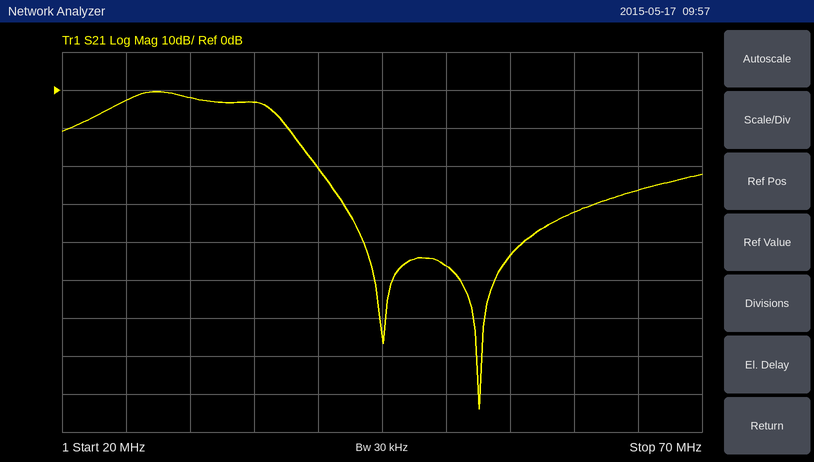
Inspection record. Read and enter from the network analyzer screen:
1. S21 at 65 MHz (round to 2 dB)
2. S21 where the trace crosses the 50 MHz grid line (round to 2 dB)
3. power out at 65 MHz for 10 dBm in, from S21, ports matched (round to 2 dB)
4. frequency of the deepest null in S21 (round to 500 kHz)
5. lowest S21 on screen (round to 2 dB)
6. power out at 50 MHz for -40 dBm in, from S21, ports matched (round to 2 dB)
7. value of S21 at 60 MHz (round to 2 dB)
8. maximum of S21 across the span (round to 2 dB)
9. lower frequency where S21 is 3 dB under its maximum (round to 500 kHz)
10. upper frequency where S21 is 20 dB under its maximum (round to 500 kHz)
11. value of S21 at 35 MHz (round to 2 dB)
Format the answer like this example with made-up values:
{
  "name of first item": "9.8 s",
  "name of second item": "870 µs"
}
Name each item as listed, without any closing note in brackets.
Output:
{
  "S21 at 65 MHz": "-26 dB",
  "S21 where the trace crosses the 50 MHz grid line": "-46 dB",
  "power out at 65 MHz for 10 dBm in, from S21, ports matched": "-16 dBm",
  "frequency of the deepest null in S21": "52.5 MHz",
  "lowest S21 on screen": "-84 dB",
  "power out at 50 MHz for -40 dBm in, from S21, ports matched": "-86 dBm",
  "value of S21 at 60 MHz": "-32 dB",
  "maximum of S21 across the span": "0 dB",
  "lower frequency where S21 is 3 dB under its maximum": "24.5 MHz",
  "upper frequency where S21 is 20 dB under its maximum": "40.0 MHz",
  "value of S21 at 35 MHz": "-4 dB"
}
